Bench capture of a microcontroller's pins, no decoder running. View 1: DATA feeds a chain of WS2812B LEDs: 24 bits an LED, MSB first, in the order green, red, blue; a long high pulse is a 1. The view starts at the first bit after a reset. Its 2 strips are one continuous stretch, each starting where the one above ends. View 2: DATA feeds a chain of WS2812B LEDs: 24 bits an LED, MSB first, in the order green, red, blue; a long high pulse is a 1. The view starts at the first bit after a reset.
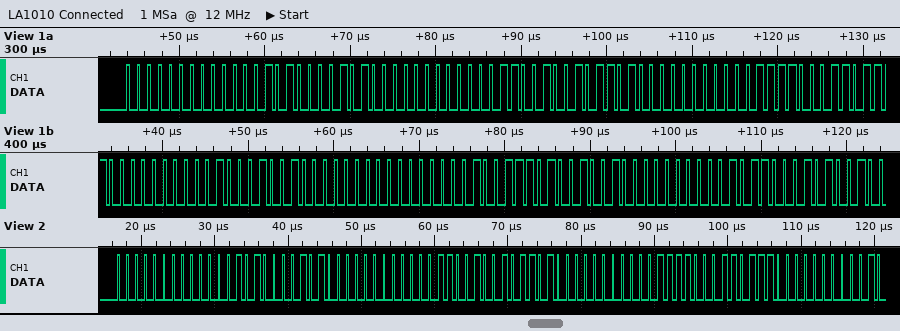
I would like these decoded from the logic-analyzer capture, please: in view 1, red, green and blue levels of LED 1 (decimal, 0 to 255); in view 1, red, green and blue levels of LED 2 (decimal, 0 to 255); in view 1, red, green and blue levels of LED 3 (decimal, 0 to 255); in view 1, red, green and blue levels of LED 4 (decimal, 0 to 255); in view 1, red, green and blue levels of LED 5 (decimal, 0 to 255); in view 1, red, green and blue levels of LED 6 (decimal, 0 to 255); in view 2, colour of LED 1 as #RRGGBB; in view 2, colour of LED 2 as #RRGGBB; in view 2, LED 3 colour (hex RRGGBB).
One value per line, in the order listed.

5, 0, 10
25, 0, 45
30, 0, 55
34, 0, 64
39, 0, 73
44, 0, 82
#05000A
#19002D
#1E0037
